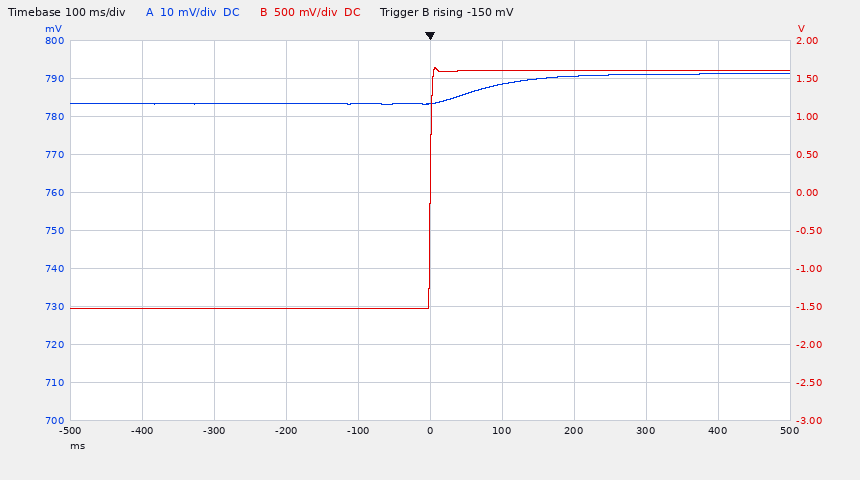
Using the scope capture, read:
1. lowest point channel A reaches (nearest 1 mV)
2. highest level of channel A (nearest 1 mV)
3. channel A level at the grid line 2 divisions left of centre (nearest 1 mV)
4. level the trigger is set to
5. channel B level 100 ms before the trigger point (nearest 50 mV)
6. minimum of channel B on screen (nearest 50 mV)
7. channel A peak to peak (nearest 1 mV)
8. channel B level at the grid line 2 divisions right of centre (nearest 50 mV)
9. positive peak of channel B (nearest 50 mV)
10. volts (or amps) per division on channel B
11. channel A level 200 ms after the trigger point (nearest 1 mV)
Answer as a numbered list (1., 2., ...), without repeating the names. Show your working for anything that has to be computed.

1. 783 mV
2. 791 mV
3. 783 mV
4. -150 mV
5. -1.55 V
6. -1.55 V
7. 791 mV − (783 mV) = 8 mV
8. 1.60 V
9. 1.65 V
10. 500 mV
11. 791 mV
